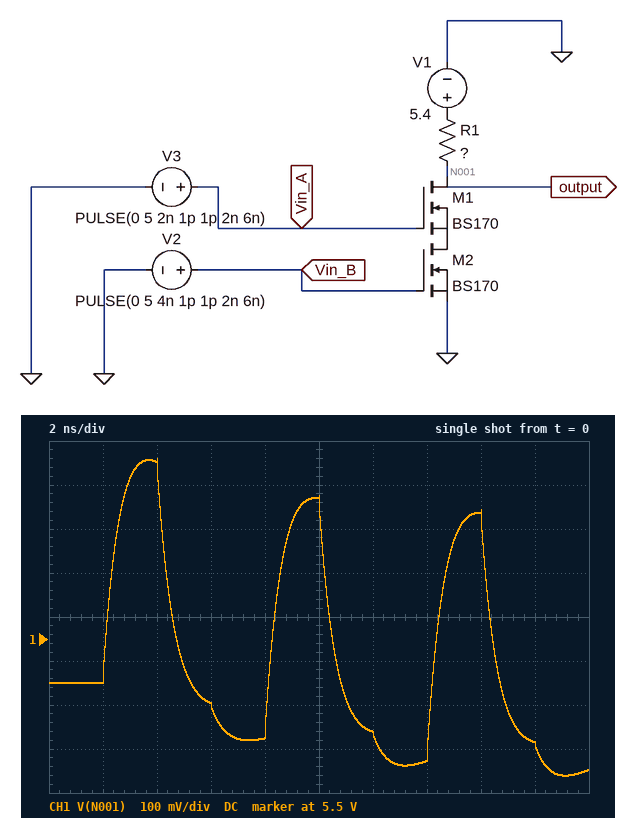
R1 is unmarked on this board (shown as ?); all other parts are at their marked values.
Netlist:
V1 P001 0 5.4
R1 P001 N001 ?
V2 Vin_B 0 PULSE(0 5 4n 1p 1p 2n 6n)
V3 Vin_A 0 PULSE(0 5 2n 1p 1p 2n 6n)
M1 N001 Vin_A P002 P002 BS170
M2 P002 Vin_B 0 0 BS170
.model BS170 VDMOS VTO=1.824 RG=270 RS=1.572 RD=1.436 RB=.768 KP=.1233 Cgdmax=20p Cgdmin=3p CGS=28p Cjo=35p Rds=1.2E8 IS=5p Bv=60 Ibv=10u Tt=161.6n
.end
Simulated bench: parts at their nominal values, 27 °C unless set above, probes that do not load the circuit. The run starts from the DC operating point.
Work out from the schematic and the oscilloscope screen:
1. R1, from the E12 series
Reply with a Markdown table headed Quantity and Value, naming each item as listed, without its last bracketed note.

| Quantity | Value |
|---|---|
| R1, from the E12 series | 68 Ω |
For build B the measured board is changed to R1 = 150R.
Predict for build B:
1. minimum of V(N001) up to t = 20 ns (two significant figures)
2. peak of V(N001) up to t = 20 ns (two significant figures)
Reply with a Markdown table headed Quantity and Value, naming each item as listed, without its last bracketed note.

| Quantity | Value |
|---|---|
| minimum of V(N001) up to t = 20 ns | 5.1 V |
| peak of V(N001) up to t = 20 ns | 6.3 V |
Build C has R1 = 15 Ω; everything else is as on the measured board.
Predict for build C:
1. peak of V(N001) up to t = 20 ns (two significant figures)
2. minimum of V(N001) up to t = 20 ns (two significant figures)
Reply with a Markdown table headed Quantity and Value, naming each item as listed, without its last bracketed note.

| Quantity | Value |
|---|---|
| peak of V(N001) up to t = 20 ns | 5.5 V |
| minimum of V(N001) up to t = 20 ns | 5.3 V |
